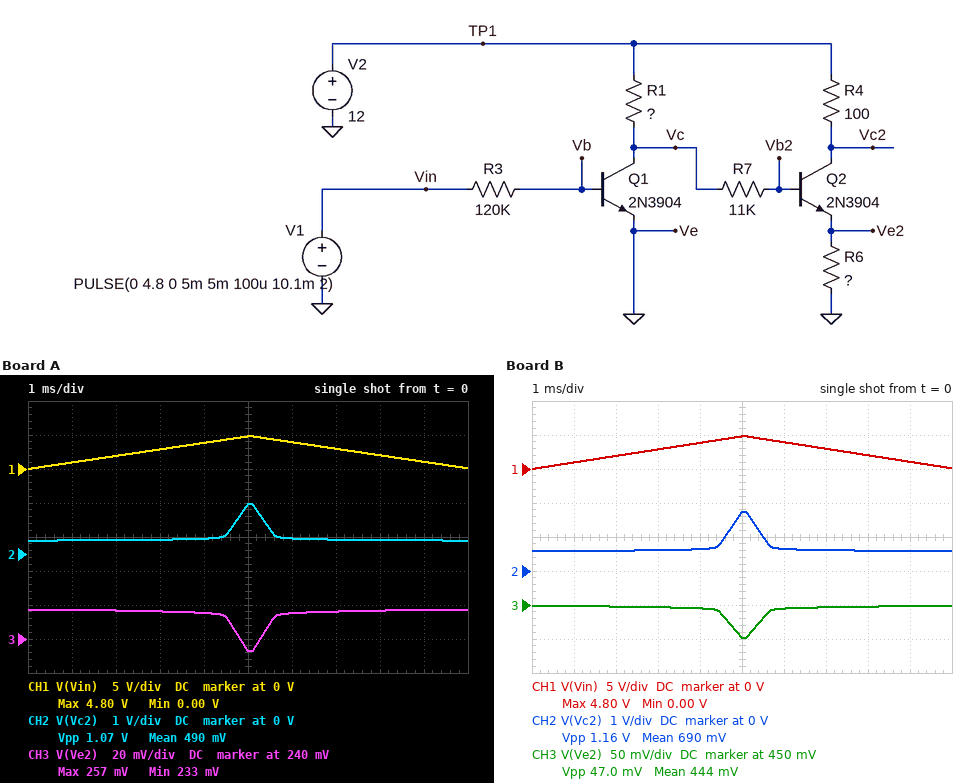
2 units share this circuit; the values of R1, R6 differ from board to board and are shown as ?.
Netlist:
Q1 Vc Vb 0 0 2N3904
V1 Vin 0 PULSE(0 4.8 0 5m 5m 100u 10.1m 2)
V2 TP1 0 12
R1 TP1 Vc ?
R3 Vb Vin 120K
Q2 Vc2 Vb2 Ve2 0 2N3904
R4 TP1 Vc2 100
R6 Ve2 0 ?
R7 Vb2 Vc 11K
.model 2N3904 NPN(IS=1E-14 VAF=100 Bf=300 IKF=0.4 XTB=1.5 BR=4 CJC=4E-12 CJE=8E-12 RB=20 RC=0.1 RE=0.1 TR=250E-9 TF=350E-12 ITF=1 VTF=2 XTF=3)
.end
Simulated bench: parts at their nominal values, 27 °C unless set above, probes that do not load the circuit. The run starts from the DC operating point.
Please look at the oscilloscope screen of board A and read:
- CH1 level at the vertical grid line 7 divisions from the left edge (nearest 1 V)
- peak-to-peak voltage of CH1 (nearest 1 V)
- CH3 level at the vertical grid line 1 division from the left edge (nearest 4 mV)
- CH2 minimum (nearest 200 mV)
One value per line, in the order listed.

3 V
5 V
256 mV
400 mV
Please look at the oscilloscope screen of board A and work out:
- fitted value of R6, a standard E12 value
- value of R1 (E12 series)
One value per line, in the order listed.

2.2 Ω
560 Ω
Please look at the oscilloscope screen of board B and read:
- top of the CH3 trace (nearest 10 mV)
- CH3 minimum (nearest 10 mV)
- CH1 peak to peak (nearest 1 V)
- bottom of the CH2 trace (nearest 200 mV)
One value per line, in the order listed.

450 mV
400 mV
5 V
600 mV
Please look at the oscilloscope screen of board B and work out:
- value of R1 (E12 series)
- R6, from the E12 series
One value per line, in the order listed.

560 Ω
3.9 Ω
